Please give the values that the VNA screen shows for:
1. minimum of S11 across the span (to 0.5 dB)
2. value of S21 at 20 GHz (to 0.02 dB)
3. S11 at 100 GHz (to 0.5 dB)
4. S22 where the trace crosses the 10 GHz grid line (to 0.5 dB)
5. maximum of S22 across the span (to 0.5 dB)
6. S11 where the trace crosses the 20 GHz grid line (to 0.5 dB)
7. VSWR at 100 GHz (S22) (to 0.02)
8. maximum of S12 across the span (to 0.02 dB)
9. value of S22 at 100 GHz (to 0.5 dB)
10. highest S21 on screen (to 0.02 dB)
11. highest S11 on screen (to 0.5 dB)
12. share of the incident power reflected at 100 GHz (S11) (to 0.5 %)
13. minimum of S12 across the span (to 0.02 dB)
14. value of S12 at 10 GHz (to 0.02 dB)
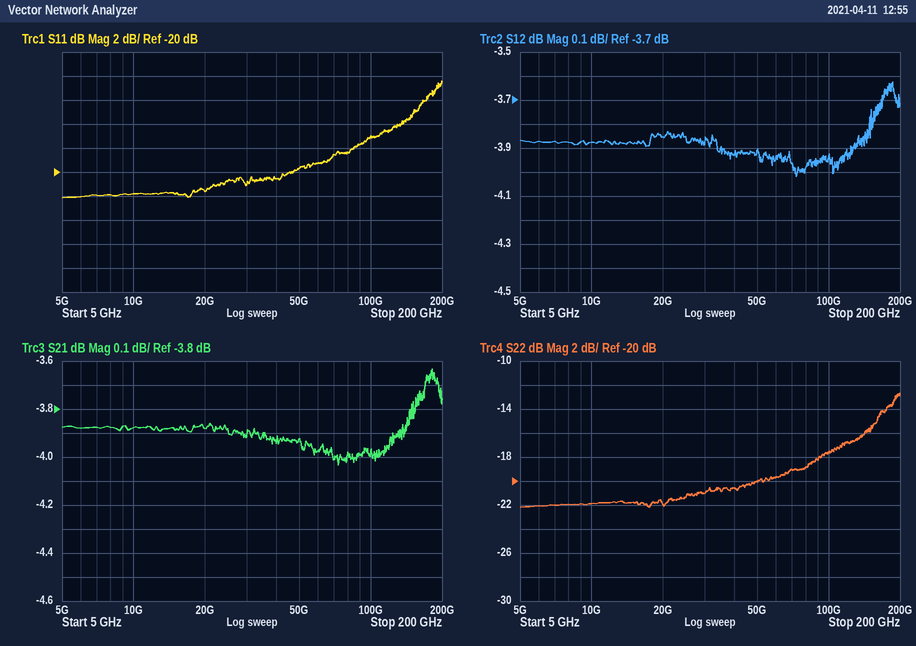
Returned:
-22.0 dB
-3.88 dB
-17.0 dB
-22.0 dB
-12.5 dB
-21.5 dB
1.30
-3.62 dB
-17.5 dB
-3.64 dB
-12.5 dB
2.0 %
-4.02 dB
-3.88 dB
